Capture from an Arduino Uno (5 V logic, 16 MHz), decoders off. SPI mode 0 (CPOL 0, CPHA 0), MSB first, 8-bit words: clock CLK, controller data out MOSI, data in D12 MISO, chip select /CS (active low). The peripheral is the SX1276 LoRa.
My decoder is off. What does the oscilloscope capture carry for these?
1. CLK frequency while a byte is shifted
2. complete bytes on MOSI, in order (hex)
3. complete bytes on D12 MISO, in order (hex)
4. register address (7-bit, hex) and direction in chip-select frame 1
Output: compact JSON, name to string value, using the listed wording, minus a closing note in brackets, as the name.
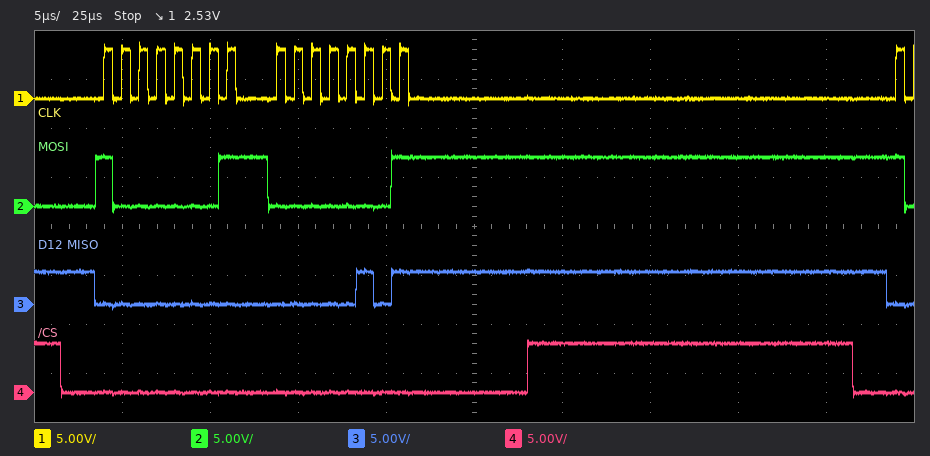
{"CLK frequency while a byte is shifted": "1 MHz", "complete bytes on MOSI, in order": "0x81 0x01", "complete bytes on D12 MISO, in order": "0x00 0x05", "register address (7-bit, hex) and direction in chip-select frame 1": "0x01 write"}
